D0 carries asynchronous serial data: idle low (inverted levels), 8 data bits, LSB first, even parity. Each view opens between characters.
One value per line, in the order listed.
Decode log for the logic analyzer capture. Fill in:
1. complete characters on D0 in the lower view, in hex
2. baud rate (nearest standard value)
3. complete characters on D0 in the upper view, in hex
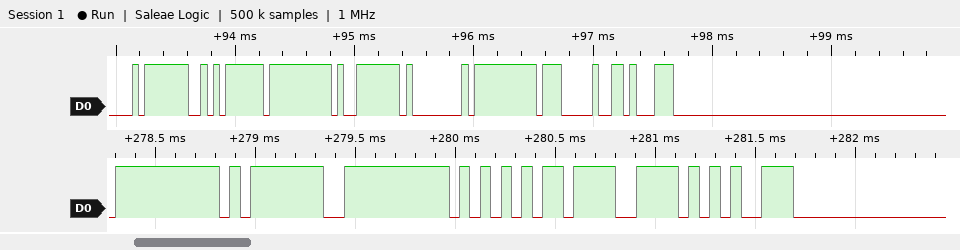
00, 01, 00, 55, 18, 35
19200 baud
01, 05, 00, 03, FF, 00, 7C, 3A
